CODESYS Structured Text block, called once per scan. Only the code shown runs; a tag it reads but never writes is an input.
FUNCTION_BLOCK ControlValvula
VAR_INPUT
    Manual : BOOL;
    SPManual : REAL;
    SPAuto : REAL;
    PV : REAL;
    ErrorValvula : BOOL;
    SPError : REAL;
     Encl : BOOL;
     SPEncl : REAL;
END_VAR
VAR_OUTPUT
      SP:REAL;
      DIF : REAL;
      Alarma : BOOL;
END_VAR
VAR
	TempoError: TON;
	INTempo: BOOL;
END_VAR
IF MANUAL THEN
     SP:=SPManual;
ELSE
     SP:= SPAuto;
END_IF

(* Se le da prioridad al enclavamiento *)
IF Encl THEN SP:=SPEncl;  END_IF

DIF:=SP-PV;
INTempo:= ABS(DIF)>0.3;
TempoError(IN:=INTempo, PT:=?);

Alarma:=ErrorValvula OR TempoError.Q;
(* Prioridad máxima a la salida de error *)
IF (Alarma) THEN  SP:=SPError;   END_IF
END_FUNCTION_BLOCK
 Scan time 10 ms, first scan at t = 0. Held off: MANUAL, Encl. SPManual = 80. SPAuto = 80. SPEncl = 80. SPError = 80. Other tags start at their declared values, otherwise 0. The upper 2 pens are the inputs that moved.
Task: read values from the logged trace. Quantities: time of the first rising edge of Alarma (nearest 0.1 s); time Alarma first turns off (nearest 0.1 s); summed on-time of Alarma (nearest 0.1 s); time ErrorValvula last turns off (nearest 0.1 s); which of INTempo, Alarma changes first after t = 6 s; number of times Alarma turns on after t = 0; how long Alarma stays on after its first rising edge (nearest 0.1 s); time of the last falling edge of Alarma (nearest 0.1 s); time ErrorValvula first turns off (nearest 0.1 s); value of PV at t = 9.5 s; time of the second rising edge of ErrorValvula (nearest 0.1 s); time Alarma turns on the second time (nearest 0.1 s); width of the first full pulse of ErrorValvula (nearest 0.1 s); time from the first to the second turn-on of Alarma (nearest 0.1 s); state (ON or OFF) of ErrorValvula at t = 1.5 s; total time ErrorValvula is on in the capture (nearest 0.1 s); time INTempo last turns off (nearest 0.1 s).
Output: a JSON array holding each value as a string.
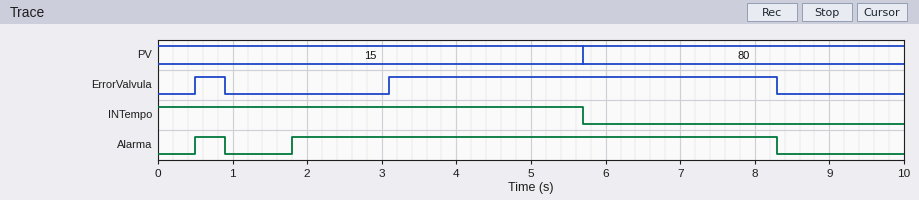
["0.5 s", "0.9 s", "6.9 s", "8.3 s", "Alarma", "2", "0.4 s", "8.3 s", "0.9 s", "80", "3.1 s", "1.8 s", "0.4 s", "1.3 s", "OFF", "5.6 s", "5.7 s"]
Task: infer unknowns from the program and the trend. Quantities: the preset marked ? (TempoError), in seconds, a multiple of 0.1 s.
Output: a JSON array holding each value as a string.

["1.8 s"]
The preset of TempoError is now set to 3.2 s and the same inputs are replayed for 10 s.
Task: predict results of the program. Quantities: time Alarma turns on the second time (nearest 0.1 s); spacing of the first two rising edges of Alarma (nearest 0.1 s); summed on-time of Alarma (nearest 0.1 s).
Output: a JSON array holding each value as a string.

["3.1 s", "2.6 s", "5.6 s"]
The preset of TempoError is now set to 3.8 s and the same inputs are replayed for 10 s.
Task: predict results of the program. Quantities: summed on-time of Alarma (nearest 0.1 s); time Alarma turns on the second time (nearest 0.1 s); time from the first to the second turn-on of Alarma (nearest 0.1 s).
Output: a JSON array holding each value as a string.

["5.6 s", "3.1 s", "2.6 s"]
